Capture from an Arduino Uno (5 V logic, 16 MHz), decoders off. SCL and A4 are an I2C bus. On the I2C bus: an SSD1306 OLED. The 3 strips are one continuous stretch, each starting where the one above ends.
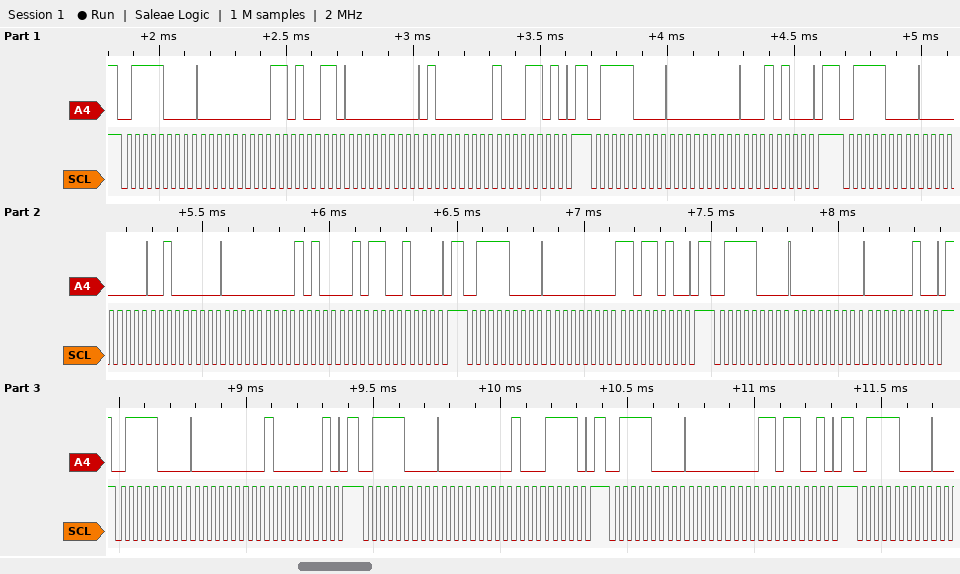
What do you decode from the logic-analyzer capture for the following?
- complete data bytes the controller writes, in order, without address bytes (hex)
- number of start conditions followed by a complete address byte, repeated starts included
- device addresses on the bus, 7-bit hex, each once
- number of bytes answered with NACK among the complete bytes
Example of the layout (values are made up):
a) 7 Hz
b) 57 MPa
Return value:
a) 00 D3 00 40 8D 00 14 00 20 00 A1 C8 00 DA 00 02 00 81 00 8F 00 D9
b) 9
c) 0x3C
d) 0
